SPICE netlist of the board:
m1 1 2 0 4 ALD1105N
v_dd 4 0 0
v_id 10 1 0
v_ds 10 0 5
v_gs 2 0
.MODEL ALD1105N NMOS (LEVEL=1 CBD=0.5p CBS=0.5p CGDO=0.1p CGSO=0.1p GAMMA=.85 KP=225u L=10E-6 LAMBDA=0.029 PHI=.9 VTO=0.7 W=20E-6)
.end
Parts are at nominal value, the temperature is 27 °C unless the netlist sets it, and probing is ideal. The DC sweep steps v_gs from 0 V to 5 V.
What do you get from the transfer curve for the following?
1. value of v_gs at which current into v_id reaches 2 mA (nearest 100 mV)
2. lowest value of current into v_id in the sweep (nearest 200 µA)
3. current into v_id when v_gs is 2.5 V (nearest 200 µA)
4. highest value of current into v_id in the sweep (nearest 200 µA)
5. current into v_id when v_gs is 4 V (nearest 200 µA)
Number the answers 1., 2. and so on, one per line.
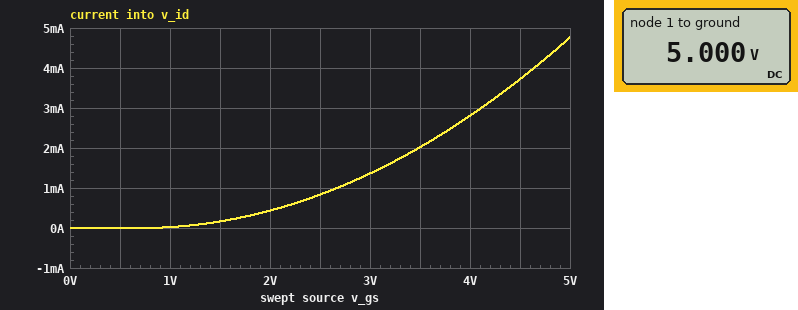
1. 3.5 V
2. 0 A
3. 800 µA
4. 4.8 mA
5. 2.8 mA
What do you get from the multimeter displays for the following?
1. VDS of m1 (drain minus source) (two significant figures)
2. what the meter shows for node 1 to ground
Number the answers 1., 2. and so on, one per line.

1. 5.0 V
2. 5.000 V
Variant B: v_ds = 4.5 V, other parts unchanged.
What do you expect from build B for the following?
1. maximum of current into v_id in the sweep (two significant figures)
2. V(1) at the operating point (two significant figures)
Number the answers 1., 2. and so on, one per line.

1. 4.7 mA
2. 4.5 V
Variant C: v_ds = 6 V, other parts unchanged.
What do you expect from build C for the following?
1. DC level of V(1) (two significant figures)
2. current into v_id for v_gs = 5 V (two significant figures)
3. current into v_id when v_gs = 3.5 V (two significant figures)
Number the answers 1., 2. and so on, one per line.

1. 6.0 V
2. 4.9 mA
3. 2.1 mA
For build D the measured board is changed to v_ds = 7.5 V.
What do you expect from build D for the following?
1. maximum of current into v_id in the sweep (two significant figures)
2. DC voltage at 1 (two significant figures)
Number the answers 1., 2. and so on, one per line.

1. 5.1 mA
2. 7.5 V
